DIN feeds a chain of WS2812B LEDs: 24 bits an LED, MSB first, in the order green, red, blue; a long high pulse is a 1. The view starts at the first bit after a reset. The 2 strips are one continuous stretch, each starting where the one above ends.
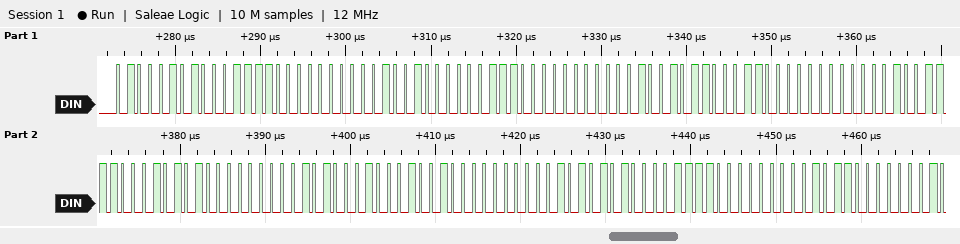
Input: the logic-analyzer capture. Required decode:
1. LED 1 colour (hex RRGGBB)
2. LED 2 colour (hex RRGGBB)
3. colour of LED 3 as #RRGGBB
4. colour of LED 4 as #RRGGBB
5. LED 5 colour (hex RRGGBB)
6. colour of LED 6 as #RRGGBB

#1E4500
#1C4800
#184B00
#154F00
#125100
#0F5500
